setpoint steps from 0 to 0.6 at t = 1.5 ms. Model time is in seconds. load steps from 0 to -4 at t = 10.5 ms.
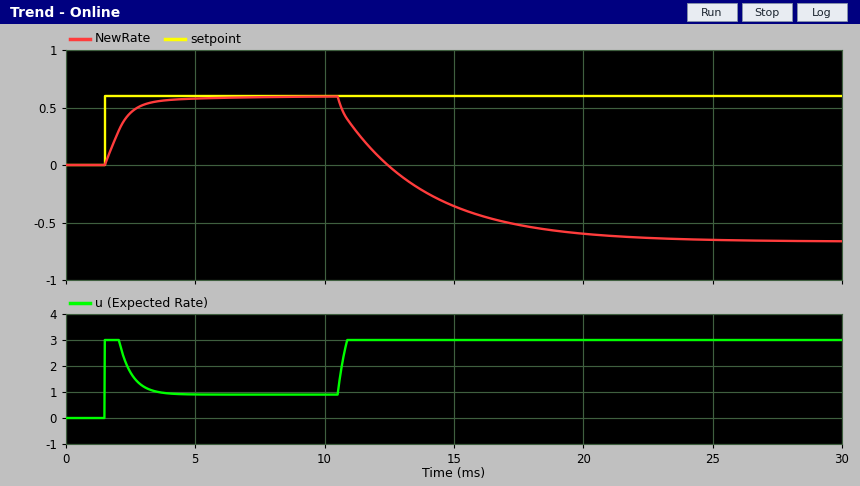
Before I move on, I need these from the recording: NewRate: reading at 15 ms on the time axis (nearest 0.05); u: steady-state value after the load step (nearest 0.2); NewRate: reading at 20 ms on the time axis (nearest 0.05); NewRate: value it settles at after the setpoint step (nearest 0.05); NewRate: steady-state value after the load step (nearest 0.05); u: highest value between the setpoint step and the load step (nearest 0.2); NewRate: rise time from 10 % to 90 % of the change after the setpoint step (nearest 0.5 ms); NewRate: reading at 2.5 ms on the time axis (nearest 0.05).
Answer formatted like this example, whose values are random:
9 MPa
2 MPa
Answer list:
-0.35
3.0
-0.60
0.60
-0.65
3.0
1.5 ms
0.45
